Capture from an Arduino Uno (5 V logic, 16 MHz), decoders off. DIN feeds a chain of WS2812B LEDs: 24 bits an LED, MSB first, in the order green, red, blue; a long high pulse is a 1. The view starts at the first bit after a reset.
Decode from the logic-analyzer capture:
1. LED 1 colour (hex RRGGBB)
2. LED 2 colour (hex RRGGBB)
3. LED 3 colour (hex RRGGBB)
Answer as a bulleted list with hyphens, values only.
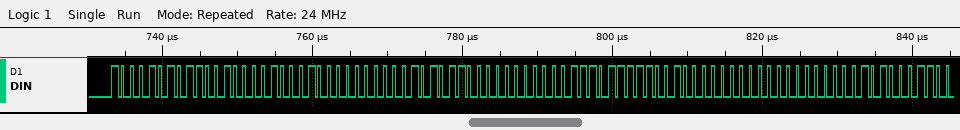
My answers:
- #C88A44
- #AC0000
- #C87700
